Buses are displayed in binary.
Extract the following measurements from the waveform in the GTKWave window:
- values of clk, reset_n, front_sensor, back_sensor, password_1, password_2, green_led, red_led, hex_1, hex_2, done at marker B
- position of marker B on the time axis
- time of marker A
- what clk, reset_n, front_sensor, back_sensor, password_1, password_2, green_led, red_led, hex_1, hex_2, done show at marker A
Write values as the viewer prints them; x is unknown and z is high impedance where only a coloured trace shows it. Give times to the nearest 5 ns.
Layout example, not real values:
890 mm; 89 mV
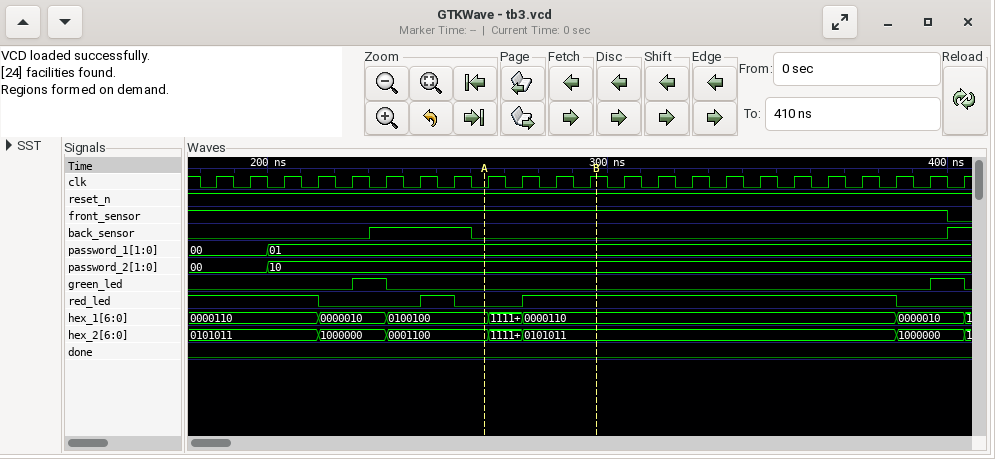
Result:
clk=1, reset_n=1, front_sensor=1, back_sensor=0, password_1=01, password_2=10, green_led=0, red_led=1, hex_1=0000110, hex_2=0101011, done=0; 295 ns; 265 ns; clk=0, reset_n=1, front_sensor=1, back_sensor=0, password_1=01, password_2=10, green_led=0, red_led=0, hex_1=0100100, hex_2=0001100, done=0
